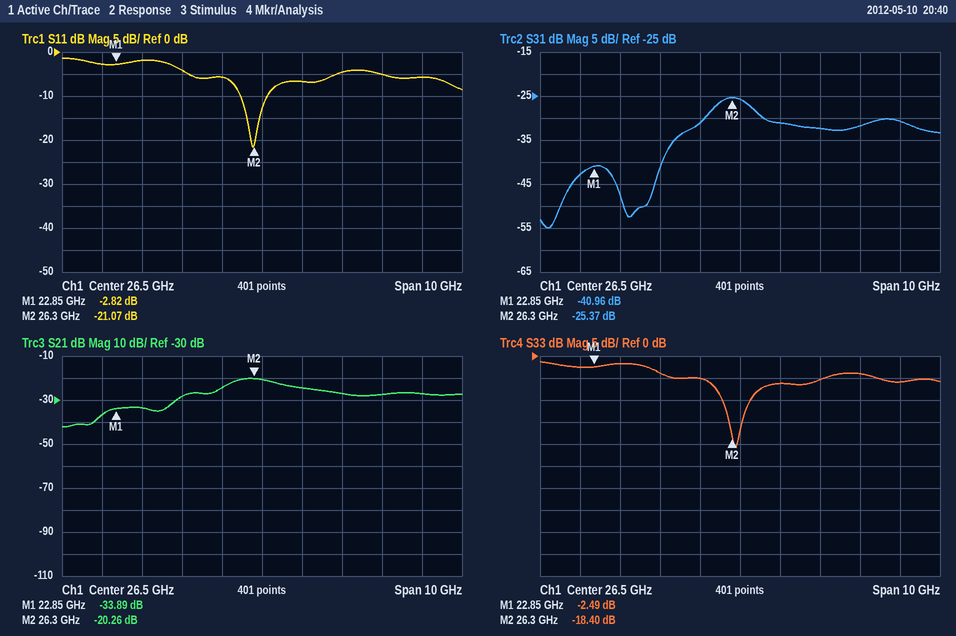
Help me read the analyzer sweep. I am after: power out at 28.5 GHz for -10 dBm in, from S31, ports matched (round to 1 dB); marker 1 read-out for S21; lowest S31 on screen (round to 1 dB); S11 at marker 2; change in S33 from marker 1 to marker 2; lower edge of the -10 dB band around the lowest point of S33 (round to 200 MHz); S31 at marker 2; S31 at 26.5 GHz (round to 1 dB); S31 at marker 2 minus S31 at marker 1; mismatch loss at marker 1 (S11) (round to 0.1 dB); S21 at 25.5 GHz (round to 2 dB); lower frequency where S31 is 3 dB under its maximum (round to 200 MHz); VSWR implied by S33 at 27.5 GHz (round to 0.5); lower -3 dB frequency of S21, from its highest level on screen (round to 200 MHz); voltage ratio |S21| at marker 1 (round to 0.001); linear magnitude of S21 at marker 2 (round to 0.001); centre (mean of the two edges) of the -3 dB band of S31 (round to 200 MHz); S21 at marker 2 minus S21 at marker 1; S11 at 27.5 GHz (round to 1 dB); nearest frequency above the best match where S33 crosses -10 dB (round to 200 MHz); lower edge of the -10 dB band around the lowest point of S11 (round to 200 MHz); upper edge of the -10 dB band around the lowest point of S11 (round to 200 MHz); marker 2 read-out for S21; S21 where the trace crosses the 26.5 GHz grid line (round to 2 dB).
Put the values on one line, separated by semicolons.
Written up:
-42 dBm; -33.89 dB; -55 dB; -21.07 dB; -15.91 dB; 26.0 GHz; -25.37 dB; -26 dB; 15.59 dB; 3.2 dB; -24 dB; 25.8 GHz; 3.0; 25.6 GHz; 0.020; 0.097; 26.4 GHz; 13.63 dB; -7 dB; 26.8 GHz; 26.0 GHz; 26.6 GHz; -20.26 dB; -20 dB
